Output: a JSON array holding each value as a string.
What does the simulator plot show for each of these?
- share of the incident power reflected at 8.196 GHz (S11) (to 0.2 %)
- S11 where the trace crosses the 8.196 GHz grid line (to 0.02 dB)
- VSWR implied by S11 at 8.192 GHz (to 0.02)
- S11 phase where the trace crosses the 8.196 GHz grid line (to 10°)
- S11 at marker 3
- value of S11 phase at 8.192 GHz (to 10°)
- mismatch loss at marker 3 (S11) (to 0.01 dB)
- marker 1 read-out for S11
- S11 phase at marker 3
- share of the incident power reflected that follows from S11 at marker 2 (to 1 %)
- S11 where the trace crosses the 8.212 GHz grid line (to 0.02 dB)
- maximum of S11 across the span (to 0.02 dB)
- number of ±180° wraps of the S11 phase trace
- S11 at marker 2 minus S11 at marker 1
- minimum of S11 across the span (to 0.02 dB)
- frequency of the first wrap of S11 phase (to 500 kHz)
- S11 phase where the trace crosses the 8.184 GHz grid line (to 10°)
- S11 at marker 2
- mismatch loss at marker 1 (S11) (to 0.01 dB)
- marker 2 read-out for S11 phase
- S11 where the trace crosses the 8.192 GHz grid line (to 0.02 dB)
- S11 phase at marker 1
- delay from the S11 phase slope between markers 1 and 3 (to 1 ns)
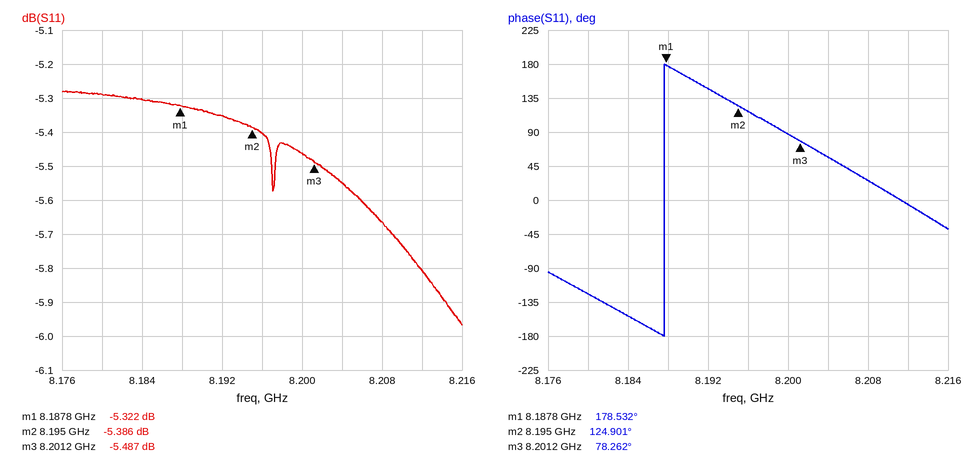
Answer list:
["28.8 %", "-5.40 dB", "3.34", "120°", "-5.487 dB", "150°", "1.44 dB", "-5.322 dB", "78.262°", "29 %", "-5.80 dB", "-5.28 dB", "1", "-0.064 dB", "-5.96 dB", "8.1875 GHz", "-150°", "-5.386 dB", "1.51 dB", "124.901°", "-5.36 dB", "178.532°", "21 ns"]
